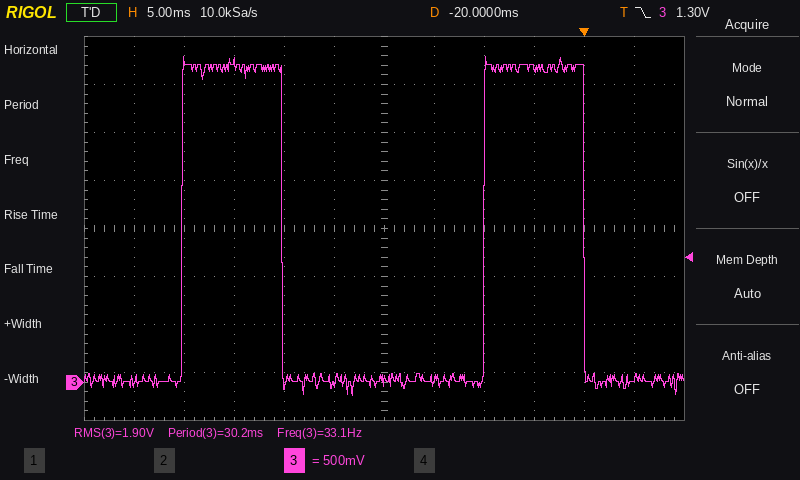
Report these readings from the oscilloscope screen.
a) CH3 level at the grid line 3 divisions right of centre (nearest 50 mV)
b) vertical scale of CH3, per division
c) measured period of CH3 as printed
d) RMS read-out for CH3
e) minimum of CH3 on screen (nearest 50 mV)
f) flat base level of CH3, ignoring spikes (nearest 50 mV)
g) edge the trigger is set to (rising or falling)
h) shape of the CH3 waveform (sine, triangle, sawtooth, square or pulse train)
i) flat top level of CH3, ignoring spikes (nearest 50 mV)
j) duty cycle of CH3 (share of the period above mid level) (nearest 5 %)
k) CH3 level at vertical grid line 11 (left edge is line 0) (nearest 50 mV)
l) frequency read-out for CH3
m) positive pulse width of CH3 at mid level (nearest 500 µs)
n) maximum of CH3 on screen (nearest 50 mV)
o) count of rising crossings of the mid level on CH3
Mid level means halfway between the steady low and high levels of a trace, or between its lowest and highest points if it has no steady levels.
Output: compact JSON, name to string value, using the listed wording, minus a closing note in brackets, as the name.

{"CH3 level at the grid line 3 divisions right of centre": "3.25 V", "vertical scale of CH3, per division": "500 mV", "measured period of CH3 as printed": "30.2 ms", "RMS read-out for CH3": "1.90 V", "minimum of CH3 on screen": "-150 mV", "flat base level of CH3, ignoring spikes": "0 mV", "edge the trigger is set to": "falling", "shape of the CH3 waveform": "pulse train", "flat top level of CH3, ignoring spikes": "3.30 V", "duty cycle of CH3 (share of the period above mid level)": "35 %", "CH3 level at vertical grid line 11 (left edge is line 0)": "50 mV", "frequency read-out for CH3": "33.1 Hz", "positive pulse width of CH3 at mid level": "10.0 ms", "maximum of CH3 on screen": "3.40 V", "count of rising crossings of the mid level on CH3": "2"}
